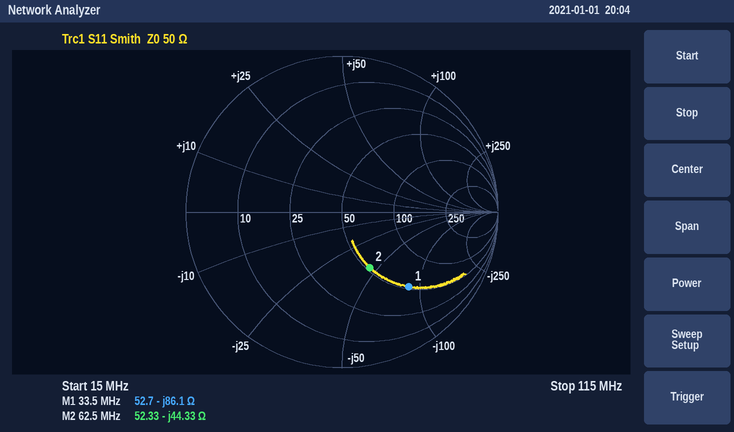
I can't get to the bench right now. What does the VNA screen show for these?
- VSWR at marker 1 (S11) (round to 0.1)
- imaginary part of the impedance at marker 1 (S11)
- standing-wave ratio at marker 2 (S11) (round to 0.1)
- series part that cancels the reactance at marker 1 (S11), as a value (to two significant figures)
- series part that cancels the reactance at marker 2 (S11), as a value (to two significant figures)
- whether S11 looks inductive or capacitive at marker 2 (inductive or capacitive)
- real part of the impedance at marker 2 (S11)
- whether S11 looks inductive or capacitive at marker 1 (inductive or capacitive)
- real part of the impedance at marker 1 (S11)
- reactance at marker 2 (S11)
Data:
4.6
-86.1 Ω
2.3
410 nH
110 nH
capacitive
52.33 Ω
capacitive
52.7 Ω
-44.33 Ω
